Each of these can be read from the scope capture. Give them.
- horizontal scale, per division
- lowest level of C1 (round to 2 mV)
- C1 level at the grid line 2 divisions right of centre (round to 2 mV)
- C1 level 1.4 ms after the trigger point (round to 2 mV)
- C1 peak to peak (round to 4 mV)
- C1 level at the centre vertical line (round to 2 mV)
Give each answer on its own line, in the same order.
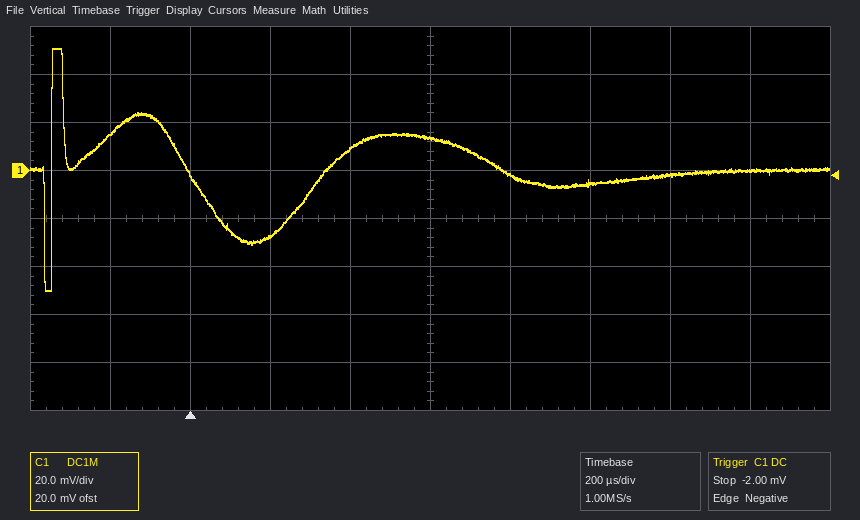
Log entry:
200 µs
-50 mV
-6 mV
0 mV
100 mV
14 mV
